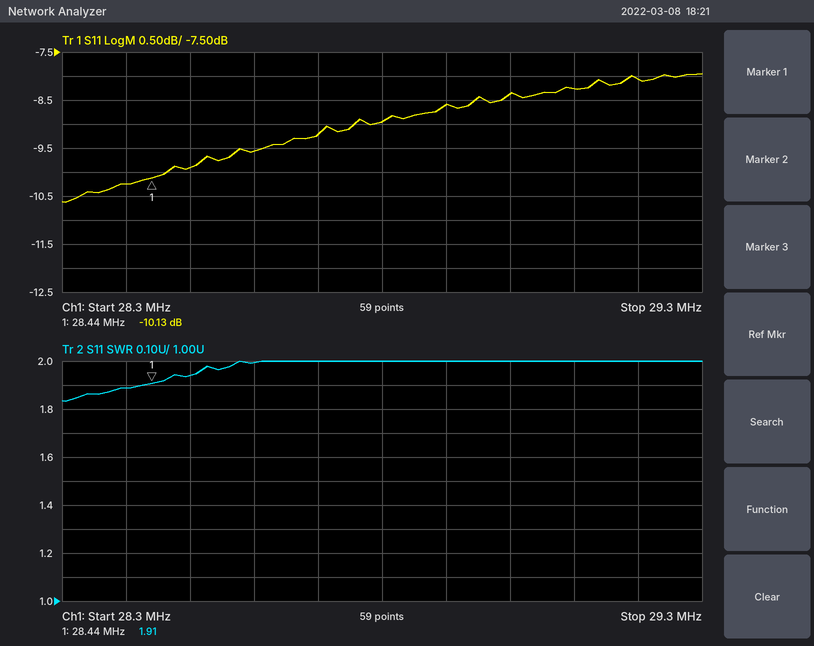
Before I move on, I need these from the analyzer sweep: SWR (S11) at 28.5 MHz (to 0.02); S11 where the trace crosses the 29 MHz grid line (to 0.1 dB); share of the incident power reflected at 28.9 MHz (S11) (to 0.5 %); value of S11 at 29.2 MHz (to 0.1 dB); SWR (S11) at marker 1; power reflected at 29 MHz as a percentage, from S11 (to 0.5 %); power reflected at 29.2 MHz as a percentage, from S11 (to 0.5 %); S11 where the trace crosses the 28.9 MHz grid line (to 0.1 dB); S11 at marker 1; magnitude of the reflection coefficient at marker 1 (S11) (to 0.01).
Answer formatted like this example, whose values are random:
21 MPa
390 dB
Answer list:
1.94
-8.4 dB
14.0 %
-8.1 dB
1.91
14.5 %
15.5 %
-8.6 dB
-10.13 dB
0.31
